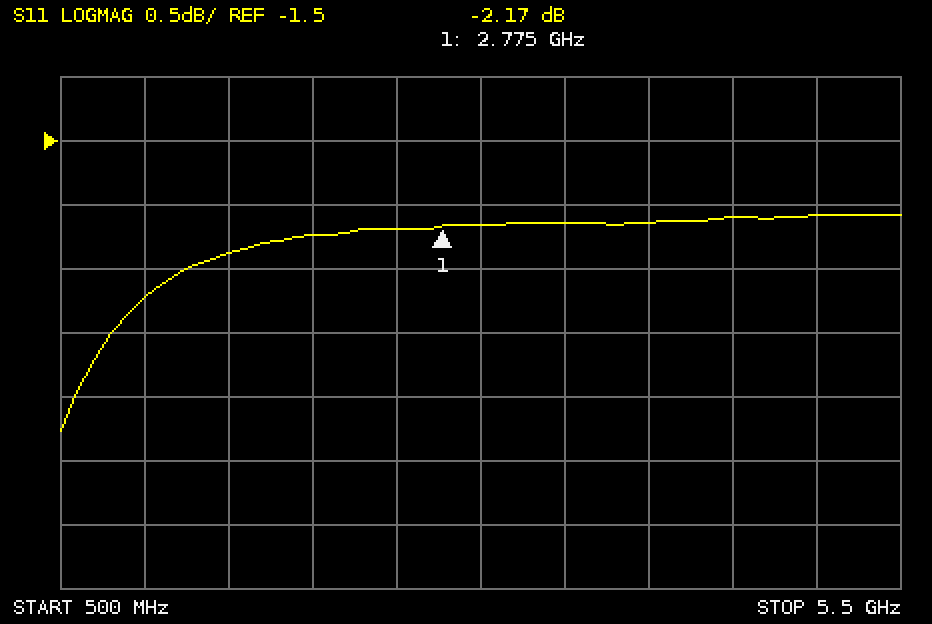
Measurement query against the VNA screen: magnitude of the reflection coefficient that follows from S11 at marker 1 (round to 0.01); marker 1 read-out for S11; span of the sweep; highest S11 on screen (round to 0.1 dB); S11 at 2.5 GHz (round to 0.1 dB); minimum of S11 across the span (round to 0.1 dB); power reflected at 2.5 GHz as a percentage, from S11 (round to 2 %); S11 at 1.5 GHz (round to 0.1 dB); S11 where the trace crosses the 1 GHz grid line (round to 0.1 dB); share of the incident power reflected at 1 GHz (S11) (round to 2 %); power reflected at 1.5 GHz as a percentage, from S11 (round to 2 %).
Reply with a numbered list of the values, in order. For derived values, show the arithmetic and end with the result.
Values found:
1. 10^(-2.17/20) ≈ 0.78
2. -2.17 dB
3. 5 GHz
4. -2.1 dB
5. -2.2 dB
6. -3.8 dB
7. 10^(-2.2/10) ≈ 60 %
8. -2.4 dB
9. -2.7 dB
10. 10^(-2.7/10) ≈ 54 %
11. 10^(-2.4/10) ≈ 58 %
